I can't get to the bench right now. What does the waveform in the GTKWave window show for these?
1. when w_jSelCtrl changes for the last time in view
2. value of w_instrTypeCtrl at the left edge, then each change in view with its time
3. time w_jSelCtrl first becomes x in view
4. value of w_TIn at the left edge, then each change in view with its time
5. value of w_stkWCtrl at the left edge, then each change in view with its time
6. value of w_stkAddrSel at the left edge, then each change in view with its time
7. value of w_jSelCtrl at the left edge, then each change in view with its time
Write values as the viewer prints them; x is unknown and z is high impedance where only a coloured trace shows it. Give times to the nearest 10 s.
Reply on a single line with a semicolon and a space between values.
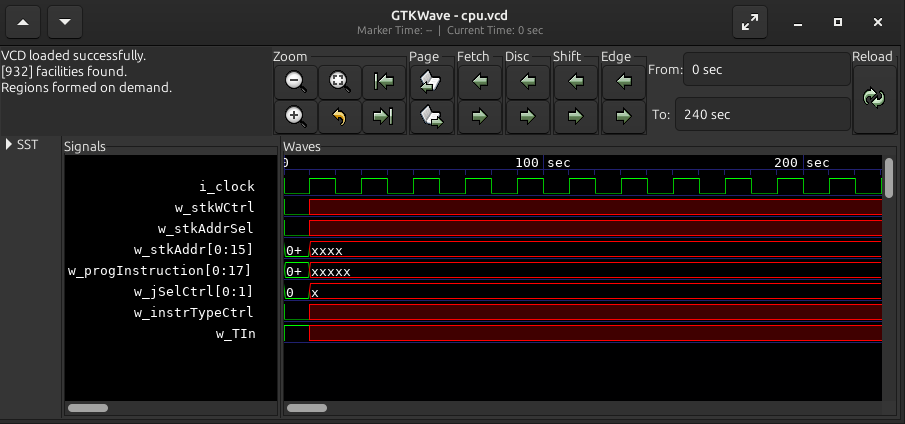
10 s; 0, x at 10 s; 10 s; 1, x at 10 s; 0, x at 10 s; 0, x at 10 s; 0, x at 10 s
